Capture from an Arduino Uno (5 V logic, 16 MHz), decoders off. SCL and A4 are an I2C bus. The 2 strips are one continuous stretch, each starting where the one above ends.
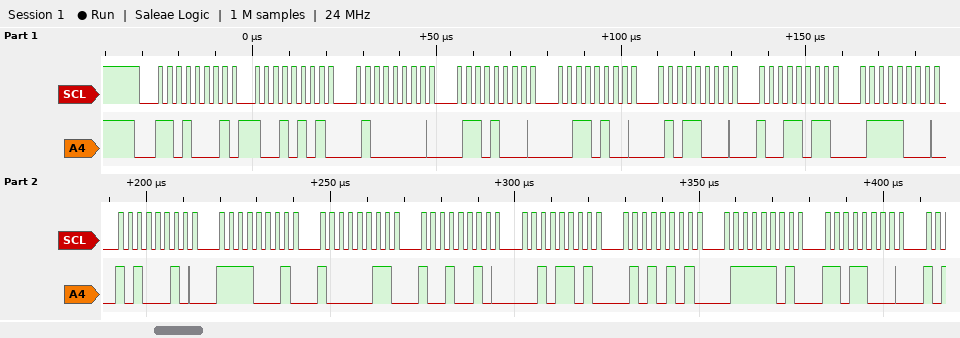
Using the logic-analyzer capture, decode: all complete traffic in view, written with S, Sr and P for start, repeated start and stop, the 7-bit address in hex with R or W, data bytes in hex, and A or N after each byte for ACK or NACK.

S 68R A 95 A 40 A 68 A 34 A 58 A 9B A 78 A A2 A F1 A 83 A 92 A 2D A 55 A 7D A D8 A
